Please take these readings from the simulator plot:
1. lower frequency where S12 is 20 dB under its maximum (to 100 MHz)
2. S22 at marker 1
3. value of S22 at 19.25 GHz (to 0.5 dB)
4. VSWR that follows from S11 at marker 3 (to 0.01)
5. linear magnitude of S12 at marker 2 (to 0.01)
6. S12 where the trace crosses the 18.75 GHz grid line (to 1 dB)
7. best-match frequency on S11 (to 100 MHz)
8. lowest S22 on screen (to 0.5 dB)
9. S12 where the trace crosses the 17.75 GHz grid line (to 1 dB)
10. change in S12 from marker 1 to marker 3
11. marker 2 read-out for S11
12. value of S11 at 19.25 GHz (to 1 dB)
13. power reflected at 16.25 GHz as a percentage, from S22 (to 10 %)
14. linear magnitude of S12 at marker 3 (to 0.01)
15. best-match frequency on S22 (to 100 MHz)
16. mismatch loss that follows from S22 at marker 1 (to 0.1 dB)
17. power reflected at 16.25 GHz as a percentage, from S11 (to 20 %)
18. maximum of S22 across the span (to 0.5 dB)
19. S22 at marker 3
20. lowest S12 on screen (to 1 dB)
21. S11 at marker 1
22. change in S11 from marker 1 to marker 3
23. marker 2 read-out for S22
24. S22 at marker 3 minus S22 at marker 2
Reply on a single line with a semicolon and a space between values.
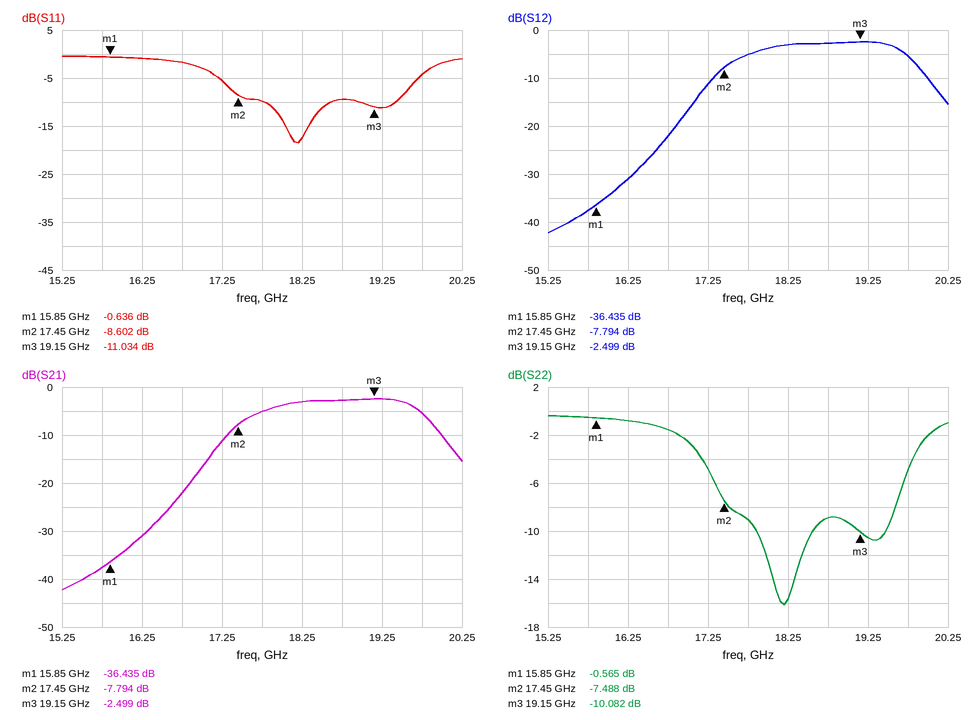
16.7 GHz; -0.565 dB; -10.5 dB; 1.78; 0.41; -3 dB; 18.2 GHz; -16.0 dB; -5 dB; 33.936 dB; -8.602 dB; -11 dB; 80 %; 0.75; 18.2 GHz; 9.1 dB; 80 %; -0.5 dB; -10.082 dB; -42 dB; -0.636 dB; -10.398 dB; -7.488 dB; -2.594 dB
